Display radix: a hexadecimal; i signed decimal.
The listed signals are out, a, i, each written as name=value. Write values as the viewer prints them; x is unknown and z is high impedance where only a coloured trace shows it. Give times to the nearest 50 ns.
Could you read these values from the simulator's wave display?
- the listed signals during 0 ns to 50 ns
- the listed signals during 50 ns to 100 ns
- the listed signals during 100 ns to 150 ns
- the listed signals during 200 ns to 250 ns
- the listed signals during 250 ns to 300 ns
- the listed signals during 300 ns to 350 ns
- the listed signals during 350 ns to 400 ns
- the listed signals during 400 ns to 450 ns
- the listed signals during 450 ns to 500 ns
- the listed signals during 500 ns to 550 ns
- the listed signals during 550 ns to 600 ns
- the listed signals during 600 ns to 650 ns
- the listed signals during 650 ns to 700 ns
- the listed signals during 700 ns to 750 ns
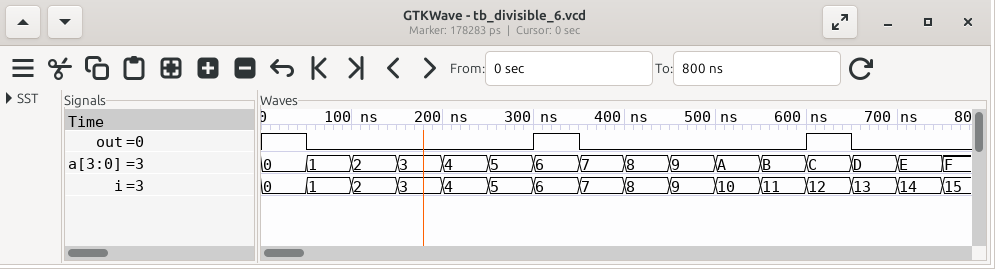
out=1, a=0, i=0
out=0, a=1, i=1
out=0, a=2, i=2
out=0, a=4, i=4
out=0, a=5, i=5
out=1, a=6, i=6
out=0, a=7, i=7
out=0, a=8, i=8
out=0, a=9, i=9
out=0, a=A, i=10
out=0, a=B, i=11
out=1, a=C, i=12
out=0, a=D, i=13
out=0, a=E, i=14
